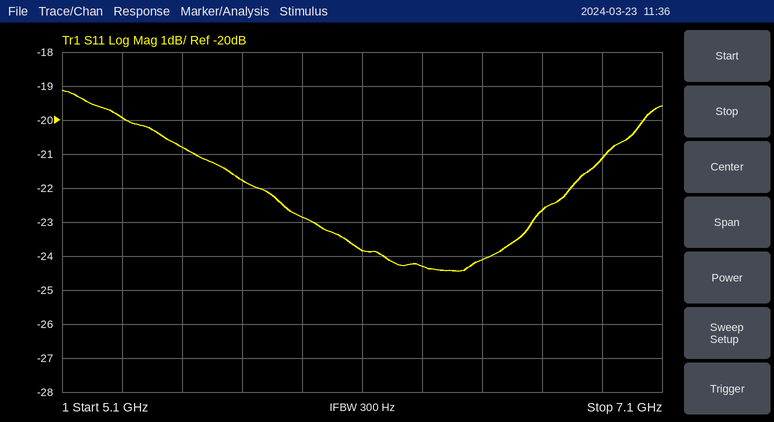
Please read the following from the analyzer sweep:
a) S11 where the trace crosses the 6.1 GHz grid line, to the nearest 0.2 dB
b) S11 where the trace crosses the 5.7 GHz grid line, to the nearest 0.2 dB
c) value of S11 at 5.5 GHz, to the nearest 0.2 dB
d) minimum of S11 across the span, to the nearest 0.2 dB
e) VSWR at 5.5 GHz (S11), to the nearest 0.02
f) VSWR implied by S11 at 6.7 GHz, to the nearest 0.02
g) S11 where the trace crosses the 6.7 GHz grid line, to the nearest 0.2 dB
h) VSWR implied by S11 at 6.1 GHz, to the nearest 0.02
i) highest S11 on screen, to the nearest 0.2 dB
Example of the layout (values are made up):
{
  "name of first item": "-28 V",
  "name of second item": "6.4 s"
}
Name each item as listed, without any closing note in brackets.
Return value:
{
  "S11 where the trace crosses the 6.1 GHz grid line, to the nearest 0.2 dB": "-23.8 dB",
  "S11 where the trace crosses the 5.7 GHz grid line, to the nearest 0.2 dB": "-21.8 dB",
  "value of S11 at 5.5 GHz, to the nearest 0.2 dB": "-20.8 dB",
  "minimum of S11 across the span, to the nearest 0.2 dB": "-24.4 dB",
  "VSWR at 5.5 GHz (S11), to the nearest 0.02": "1.20",
  "VSWR implied by S11 at 6.7 GHz, to the nearest 0.02": "1.16",
  "S11 where the trace crosses the 6.7 GHz grid line, to the nearest 0.2 dB": "-22.6 dB",
  "VSWR implied by S11 at 6.1 GHz, to the nearest 0.02": "1.14",
  "highest S11 on screen, to the nearest 0.2 dB": "-19.2 dB"
}
